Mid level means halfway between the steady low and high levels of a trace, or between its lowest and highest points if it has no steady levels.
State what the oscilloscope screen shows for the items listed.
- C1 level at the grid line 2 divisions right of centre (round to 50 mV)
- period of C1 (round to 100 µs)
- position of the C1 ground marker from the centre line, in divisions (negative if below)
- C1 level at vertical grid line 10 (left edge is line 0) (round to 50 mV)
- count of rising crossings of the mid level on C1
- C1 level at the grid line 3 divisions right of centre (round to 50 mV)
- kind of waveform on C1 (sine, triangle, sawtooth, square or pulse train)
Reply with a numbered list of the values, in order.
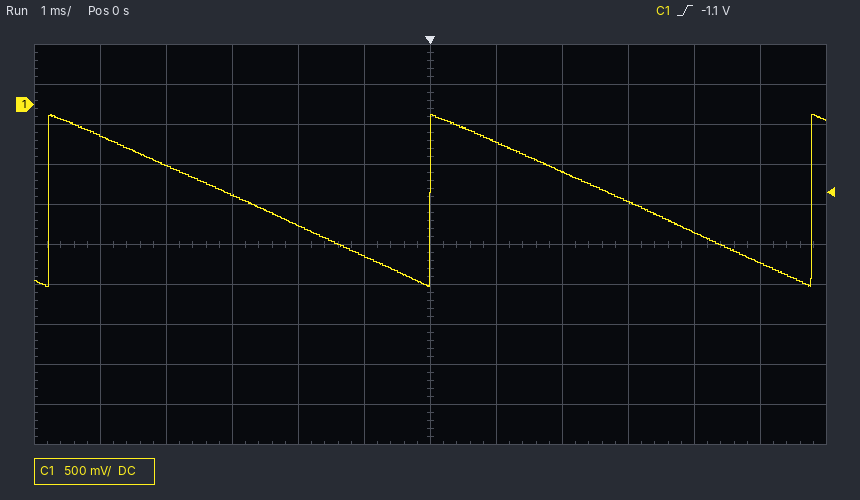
1. -850 mV
2. 5.8 ms
3. +3.5 div
4. -1.60 V
5. 3
6. -1.20 V
7. sawtooth
